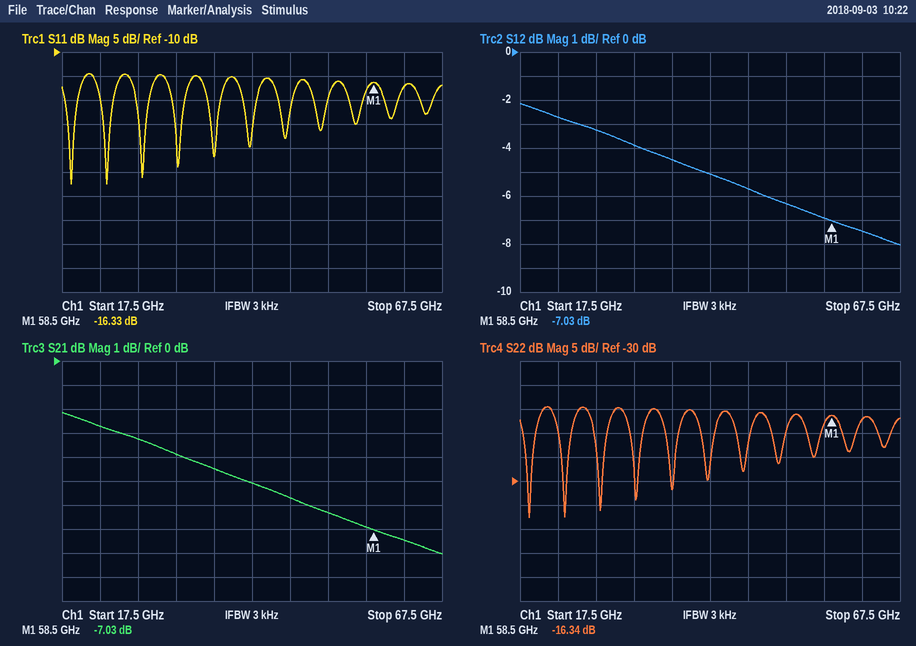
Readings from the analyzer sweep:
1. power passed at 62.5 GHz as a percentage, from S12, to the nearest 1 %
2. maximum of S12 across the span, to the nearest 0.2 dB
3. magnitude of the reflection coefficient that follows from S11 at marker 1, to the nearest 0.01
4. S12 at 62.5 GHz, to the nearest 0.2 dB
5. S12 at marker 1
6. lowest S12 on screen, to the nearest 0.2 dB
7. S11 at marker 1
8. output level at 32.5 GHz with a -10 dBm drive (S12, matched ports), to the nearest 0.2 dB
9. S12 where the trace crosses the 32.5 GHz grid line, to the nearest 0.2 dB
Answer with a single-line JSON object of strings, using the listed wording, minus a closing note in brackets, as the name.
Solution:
{"power passed at 62.5 GHz as a percentage, from S12, to the nearest 1 %": "18 %", "maximum of S12 across the span, to the nearest 0.2 dB": "-2.2 dB", "magnitude of the reflection coefficient that follows from S11 at marker 1, to the nearest 0.01": "0.15", "S12 at 62.5 GHz, to the nearest 0.2 dB": "-7.4 dB", "S12 at marker 1": "-7.03 dB", "lowest S12 on screen, to the nearest 0.2 dB": "-8.0 dB", "S11 at marker 1": "-16.33 dB", "output level at 32.5 GHz with a -10 dBm drive (S12, matched ports), to the nearest 0.2 dB": "-13.8 dBm", "S12 where the trace crosses the 32.5 GHz grid line, to the nearest 0.2 dB": "-3.8 dB"}
